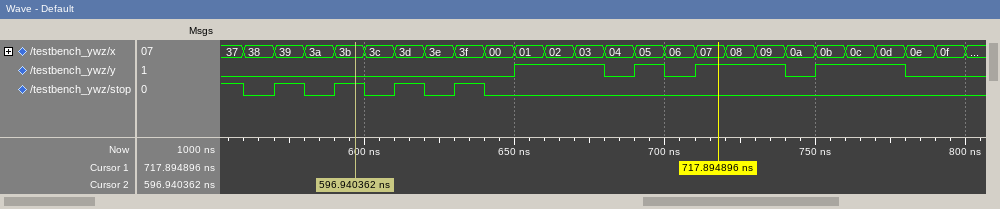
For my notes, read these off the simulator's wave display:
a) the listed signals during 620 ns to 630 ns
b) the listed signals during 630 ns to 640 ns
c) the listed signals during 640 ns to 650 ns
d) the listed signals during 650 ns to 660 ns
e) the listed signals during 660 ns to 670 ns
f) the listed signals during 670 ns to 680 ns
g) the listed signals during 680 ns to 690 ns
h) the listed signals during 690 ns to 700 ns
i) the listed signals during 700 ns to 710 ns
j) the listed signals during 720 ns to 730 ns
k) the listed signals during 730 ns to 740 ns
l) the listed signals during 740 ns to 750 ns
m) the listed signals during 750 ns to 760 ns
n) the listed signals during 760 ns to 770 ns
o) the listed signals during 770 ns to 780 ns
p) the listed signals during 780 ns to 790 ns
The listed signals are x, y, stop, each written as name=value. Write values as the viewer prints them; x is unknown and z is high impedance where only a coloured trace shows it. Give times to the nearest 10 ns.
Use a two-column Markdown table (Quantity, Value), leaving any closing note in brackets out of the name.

| Quantity | Value |
|---|---|
| the listed signals during 620 ns to 630 ns | x=3e, y=0, stop=0 |
| the listed signals during 630 ns to 640 ns | x=3f, y=0, stop=1 |
| the listed signals during 640 ns to 650 ns | x=00, y=0, stop=0 |
| the listed signals during 650 ns to 660 ns | x=01, y=1, stop=0 |
| the listed signals during 660 ns to 670 ns | x=02, y=1, stop=0 |
| the listed signals during 670 ns to 680 ns | x=03, y=1, stop=0 |
| the listed signals during 680 ns to 690 ns | x=04, y=0, stop=0 |
| the listed signals during 690 ns to 700 ns | x=05, y=1, stop=0 |
| the listed signals during 700 ns to 710 ns | x=06, y=0, stop=0 |
| the listed signals during 720 ns to 730 ns | x=08, y=1, stop=0 |
| the listed signals during 730 ns to 740 ns | x=09, y=1, stop=0 |
| the listed signals during 740 ns to 750 ns | x=0a, y=0, stop=0 |
| the listed signals during 750 ns to 760 ns | x=0b, y=1, stop=0 |
| the listed signals during 760 ns to 770 ns | x=0c, y=1, stop=0 |
| the listed signals during 770 ns to 780 ns | x=0d, y=1, stop=0 |
| the listed signals during 780 ns to 790 ns | x=0e, y=0, stop=0 |
